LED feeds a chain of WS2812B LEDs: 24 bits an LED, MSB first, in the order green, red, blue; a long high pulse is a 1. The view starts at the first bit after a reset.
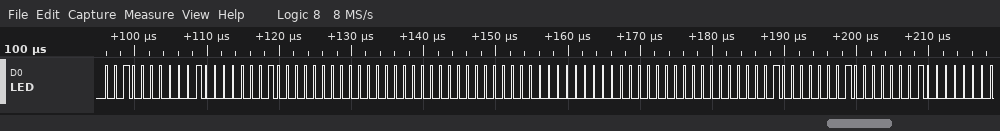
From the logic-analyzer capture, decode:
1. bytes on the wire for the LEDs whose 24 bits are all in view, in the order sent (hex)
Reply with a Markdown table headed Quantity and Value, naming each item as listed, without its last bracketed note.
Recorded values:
| Quantity | Value |
|---|---|
| bytes on the wire for the LEDs whose 24 bits are all in view, in the order sent | 20 20 20 00 00 00 00 00 00 20 20 20 |
